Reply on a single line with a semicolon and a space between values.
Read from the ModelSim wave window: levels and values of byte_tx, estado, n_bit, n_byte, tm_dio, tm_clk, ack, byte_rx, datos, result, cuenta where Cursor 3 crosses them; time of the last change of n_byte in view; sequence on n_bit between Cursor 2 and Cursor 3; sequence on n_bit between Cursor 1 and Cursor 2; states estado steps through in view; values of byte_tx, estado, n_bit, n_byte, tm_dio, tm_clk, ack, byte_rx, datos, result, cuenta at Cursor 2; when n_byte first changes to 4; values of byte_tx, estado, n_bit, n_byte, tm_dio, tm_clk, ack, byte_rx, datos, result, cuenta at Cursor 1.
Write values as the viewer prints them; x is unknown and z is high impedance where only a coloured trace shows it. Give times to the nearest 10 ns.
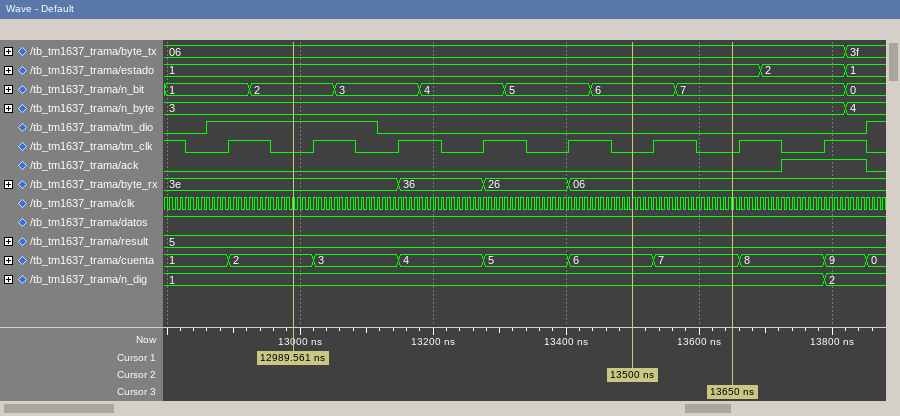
byte_tx=06, estado=1, n_bit=7, n_byte=3, tm_dio=0, tm_clk=0, ack=0, byte_rx=06, datos=1, result=5, cuenta=7; 13820 ns; 6, 7; 2, 3, 4, 5, 6; 1, 2, 1; byte_tx=06, estado=1, n_bit=6, n_byte=3, tm_dio=0, tm_clk=0, ack=0, byte_rx=06, datos=1, result=5, cuenta=6; 13820 ns; byte_tx=06, estado=1, n_bit=2, n_byte=3, tm_dio=1, tm_clk=0, ack=0, byte_rx=3e, datos=1, result=5, cuenta=2
